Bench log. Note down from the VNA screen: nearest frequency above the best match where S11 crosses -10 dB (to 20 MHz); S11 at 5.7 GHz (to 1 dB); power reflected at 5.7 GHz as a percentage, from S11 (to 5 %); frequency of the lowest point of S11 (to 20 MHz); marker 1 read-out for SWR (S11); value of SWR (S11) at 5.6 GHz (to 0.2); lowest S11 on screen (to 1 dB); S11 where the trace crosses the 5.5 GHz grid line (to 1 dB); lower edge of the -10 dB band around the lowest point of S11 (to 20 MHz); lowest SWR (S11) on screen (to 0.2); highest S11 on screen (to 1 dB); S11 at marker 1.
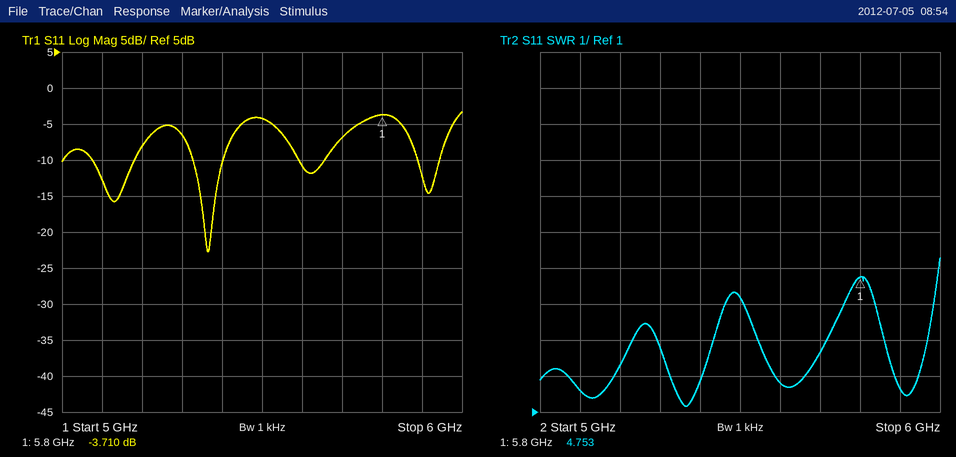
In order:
5.40 GHz
-7 dB
20 %
5.36 GHz
4.753
1.8
-23 dB
-4 dB
5.32 GHz
1.2
-3 dB
-3.710 dB
